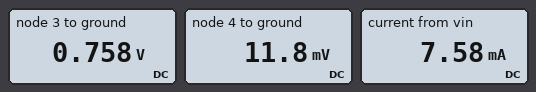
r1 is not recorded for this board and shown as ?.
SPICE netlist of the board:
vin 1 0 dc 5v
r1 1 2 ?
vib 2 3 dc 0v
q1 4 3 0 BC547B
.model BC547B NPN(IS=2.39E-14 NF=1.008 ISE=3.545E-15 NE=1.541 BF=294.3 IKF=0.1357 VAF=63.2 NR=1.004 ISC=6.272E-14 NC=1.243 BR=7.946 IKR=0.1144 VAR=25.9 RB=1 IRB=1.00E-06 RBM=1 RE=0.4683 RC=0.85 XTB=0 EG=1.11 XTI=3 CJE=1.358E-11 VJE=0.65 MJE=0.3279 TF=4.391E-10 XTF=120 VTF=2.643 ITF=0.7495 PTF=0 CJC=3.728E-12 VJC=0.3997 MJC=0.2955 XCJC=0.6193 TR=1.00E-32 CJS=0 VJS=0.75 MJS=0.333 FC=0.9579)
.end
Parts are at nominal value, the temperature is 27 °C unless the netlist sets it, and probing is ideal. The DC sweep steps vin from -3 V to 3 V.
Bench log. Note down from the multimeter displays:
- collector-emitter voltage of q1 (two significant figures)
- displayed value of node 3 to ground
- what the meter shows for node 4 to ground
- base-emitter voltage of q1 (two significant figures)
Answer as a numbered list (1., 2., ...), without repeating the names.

1. 12 mV
2. 0.758 V
3. 11.8 mV
4. 760 mV
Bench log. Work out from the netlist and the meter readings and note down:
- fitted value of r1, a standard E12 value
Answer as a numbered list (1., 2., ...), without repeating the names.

1. 560 Ω
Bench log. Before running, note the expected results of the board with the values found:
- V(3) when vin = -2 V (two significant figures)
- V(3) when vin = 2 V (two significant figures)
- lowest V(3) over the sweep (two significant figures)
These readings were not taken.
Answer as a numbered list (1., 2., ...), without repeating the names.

1. -2.0 V
2. 720 mV
3. -3.0 V
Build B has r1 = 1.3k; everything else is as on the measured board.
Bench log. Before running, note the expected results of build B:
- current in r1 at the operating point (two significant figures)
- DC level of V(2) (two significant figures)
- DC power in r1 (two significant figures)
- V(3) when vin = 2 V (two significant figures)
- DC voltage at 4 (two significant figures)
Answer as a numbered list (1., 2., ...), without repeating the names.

1. 3.3 mA
2. 730 mV
3. 14 mW
4. 690 mV
5. 8.9 mV
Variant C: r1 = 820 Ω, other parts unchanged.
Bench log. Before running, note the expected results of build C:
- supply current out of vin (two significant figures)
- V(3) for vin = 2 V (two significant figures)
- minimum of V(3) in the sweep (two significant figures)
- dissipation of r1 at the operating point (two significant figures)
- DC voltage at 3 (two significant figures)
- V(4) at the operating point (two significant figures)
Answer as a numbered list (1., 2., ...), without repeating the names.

1. 5.2 mA
2. 710 mV
3. -3.0 V
4. 22 mW
5. 740 mV
6. 10 mV
